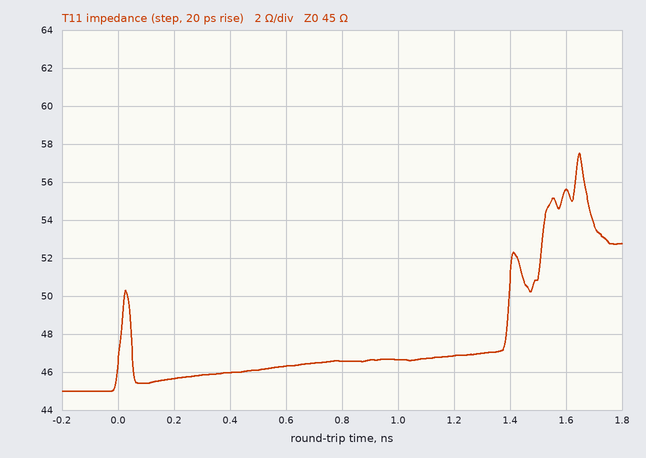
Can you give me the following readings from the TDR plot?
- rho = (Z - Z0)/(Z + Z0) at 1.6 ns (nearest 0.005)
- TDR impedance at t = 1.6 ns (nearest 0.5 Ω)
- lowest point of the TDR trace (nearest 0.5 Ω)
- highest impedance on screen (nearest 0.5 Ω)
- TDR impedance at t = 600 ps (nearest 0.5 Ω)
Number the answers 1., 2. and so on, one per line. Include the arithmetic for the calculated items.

1. (55.5 − 45)/(55.5 + 45) ≈ +0.104, so +0.105 to the nearest 0.005
2. 55.5 Ω
3. 45.0 Ω
4. 57.5 Ω
5. 46.5 Ω
